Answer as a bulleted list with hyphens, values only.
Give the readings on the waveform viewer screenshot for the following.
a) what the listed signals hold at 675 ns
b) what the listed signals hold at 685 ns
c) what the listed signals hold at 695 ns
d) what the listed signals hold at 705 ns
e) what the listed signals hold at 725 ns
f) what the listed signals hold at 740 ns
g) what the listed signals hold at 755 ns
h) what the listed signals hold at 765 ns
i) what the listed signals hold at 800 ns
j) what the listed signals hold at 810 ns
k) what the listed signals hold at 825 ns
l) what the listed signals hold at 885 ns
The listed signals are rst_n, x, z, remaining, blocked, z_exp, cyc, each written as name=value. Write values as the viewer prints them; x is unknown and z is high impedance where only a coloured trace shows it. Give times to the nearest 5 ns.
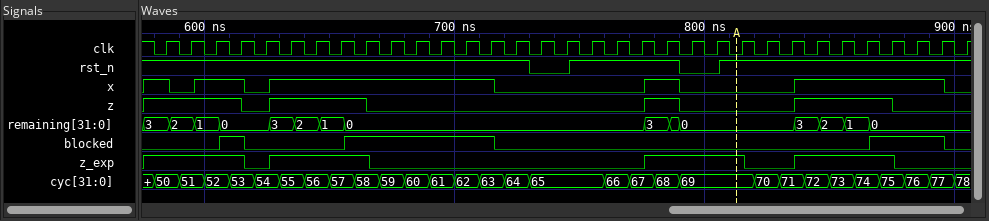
- rst_n=1, x=1, z=0, remaining=0, blocked=1, z_exp=0, cyc=59
- rst_n=1, x=1, z=0, remaining=0, blocked=1, z_exp=0, cyc=60
- rst_n=1, x=1, z=0, remaining=0, blocked=1, z_exp=0, cyc=61
- rst_n=1, x=1, z=0, remaining=0, blocked=1, z_exp=0, cyc=62
- rst_n=1, x=0, z=0, remaining=0, blocked=0, z_exp=0, cyc=64
- rst_n=0, x=0, z=0, remaining=0, blocked=0, z_exp=0, cyc=65
- rst_n=1, x=0, z=0, remaining=0, blocked=0, z_exp=0, cyc=65
- rst_n=1, x=0, z=0, remaining=0, blocked=0, z_exp=0, cyc=66
- rst_n=0, x=0, z=0, remaining=0, blocked=0, z_exp=1, cyc=69
- rst_n=1, x=0, z=0, remaining=0, blocked=0, z_exp=1, cyc=69
- rst_n=1, x=0, z=0, remaining=0, blocked=0, z_exp=0, cyc=70
- rst_n=1, x=1, z=0, remaining=0, blocked=1, z_exp=0, cyc=76
